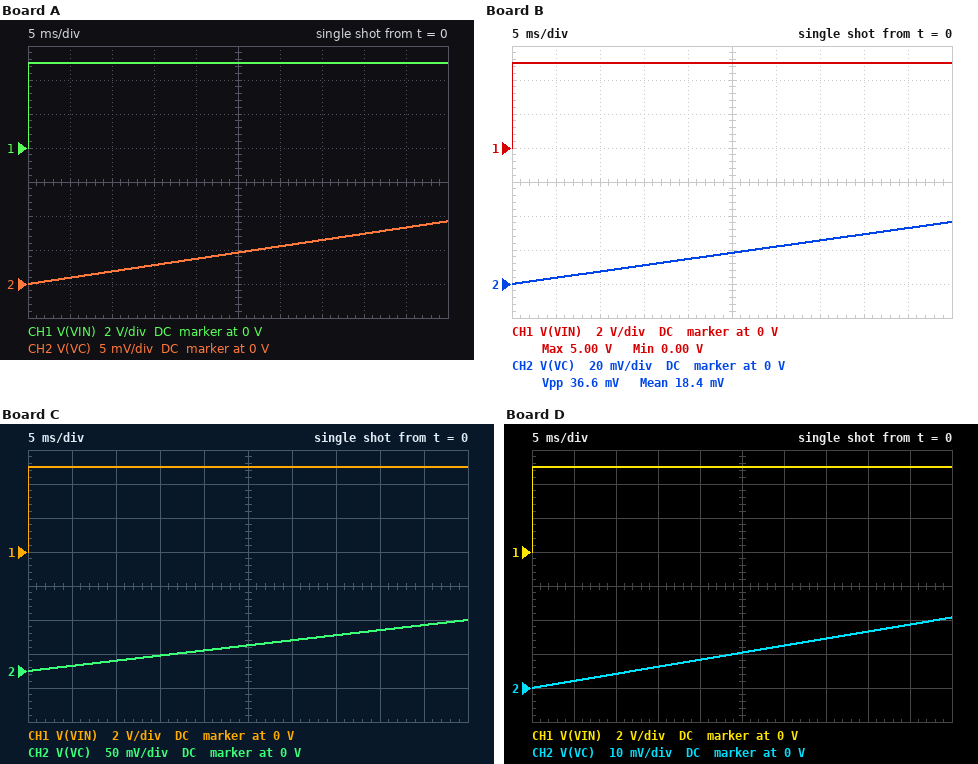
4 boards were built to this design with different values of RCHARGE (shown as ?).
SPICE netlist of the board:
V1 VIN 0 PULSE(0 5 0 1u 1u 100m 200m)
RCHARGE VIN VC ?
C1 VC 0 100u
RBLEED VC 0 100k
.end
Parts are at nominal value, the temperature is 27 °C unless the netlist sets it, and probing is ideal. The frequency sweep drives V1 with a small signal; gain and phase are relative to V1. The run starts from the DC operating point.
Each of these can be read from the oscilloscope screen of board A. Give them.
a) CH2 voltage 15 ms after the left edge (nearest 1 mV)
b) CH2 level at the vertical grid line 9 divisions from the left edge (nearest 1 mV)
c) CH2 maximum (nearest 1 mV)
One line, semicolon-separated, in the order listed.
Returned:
3 mV; 8 mV; 9 mV
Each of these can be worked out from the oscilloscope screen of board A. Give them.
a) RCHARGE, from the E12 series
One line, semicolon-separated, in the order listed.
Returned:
270 kΩ
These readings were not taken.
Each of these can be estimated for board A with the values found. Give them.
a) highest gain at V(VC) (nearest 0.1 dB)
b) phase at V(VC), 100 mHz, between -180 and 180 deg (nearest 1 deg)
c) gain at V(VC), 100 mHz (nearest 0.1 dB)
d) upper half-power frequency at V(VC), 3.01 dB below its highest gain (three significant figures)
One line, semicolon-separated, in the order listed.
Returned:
-11.4 dB; -78 deg; -24.8 dB; 21.8 mHz
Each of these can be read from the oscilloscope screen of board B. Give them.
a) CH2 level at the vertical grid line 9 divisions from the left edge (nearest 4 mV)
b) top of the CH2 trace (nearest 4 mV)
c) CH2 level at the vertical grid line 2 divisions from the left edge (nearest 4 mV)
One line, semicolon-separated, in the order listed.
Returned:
32 mV; 36 mV; 8 mV
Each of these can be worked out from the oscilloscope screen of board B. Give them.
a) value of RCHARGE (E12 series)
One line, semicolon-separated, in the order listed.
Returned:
68 kΩ
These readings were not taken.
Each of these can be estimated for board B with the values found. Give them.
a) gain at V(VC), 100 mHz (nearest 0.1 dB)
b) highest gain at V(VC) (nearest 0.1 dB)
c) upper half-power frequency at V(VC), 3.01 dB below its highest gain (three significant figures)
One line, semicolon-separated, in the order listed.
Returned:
-13.2 dB; -4.5 dB; 39.3 mHz
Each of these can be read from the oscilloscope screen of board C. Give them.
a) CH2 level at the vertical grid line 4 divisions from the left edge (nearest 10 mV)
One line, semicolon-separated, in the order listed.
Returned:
30 mV
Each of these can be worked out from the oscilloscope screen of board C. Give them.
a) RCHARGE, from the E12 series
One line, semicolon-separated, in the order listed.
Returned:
33 kΩ
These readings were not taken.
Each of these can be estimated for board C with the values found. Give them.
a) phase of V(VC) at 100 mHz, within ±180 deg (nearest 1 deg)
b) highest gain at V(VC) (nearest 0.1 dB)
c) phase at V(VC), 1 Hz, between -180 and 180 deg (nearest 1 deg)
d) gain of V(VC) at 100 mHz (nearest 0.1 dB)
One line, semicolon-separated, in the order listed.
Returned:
-57 deg; -2.5 dB; -86 deg; -7.8 dB
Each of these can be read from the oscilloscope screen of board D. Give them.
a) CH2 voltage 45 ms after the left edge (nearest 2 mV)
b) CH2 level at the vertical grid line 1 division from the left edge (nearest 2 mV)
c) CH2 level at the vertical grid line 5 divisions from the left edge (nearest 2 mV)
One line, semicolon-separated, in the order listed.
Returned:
18 mV; 2 mV; 10 mV
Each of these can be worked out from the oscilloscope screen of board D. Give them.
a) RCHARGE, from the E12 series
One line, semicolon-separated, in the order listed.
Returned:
120 kΩ
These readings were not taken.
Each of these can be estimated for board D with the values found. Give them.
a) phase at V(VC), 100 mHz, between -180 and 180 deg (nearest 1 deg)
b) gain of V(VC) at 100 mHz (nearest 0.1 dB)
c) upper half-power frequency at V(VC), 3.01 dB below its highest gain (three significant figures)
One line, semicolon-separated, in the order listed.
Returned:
-74 deg; -17.9 dB; 29.2 mHz
